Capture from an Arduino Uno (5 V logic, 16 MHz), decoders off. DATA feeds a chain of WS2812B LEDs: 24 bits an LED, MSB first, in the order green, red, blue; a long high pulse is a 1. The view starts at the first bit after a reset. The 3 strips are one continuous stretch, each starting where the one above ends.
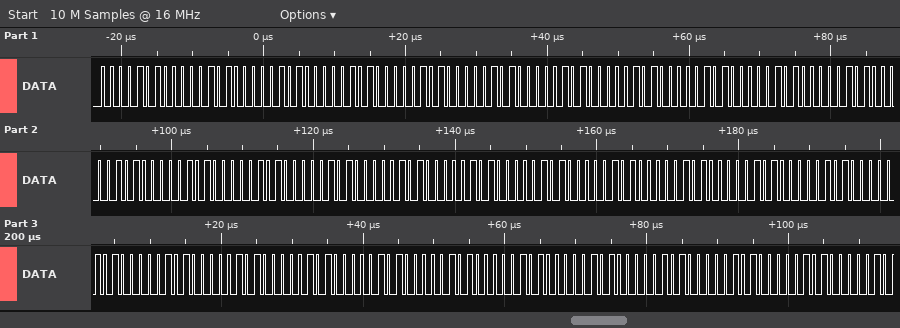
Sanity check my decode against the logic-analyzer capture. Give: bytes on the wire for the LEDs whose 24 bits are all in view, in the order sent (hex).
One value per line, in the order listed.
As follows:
0A 0A 0A 0A 0A 0A 0A 0A 0A 0A 0A 0A 0A 0A 0A 0A 0A 0A 0A 0A 0A 0A 0A 0A 0A 0A 0A 0A 0A 0A 0A 0A 0A
